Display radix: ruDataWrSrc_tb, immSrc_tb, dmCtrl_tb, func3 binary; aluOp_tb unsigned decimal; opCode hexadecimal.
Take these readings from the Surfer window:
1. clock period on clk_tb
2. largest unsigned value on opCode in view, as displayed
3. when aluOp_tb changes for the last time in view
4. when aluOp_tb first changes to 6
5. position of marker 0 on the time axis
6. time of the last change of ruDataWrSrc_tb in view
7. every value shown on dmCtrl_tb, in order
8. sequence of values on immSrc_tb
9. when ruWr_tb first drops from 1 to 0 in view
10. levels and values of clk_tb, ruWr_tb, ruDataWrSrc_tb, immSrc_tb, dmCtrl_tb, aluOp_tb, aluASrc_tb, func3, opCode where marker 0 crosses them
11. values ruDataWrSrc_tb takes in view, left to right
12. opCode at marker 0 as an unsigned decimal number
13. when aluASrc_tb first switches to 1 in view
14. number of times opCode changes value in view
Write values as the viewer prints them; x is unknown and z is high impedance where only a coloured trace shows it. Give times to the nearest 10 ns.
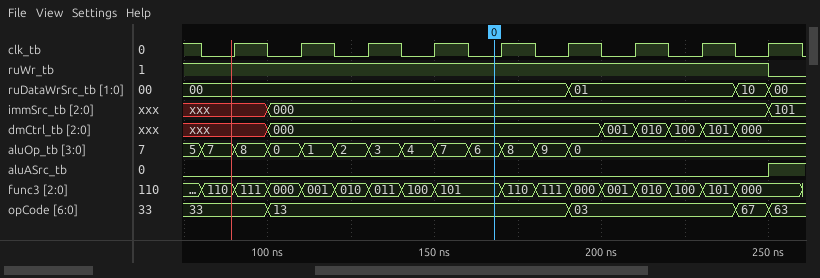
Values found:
20 ns
67
190 ns
160 ns
170 ns
250 ns
xxx, 000, 001, 010, 100, 101, 000
xxx, 000, 101
250 ns
clk_tb=0, ruWr_tb=1, ruDataWrSrc_tb=00, immSrc_tb=000, dmCtrl_tb=000, aluOp_tb=6, aluASrc_tb=0, func3=101, opCode=13
00, 01, 10, 00
19
250 ns
4
